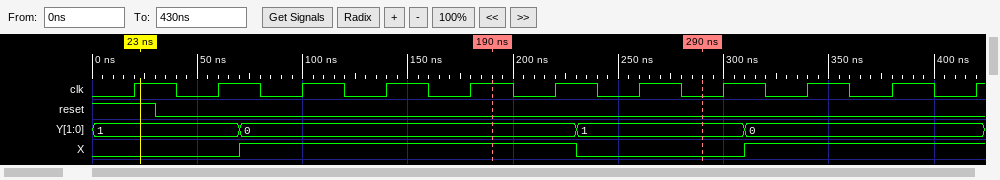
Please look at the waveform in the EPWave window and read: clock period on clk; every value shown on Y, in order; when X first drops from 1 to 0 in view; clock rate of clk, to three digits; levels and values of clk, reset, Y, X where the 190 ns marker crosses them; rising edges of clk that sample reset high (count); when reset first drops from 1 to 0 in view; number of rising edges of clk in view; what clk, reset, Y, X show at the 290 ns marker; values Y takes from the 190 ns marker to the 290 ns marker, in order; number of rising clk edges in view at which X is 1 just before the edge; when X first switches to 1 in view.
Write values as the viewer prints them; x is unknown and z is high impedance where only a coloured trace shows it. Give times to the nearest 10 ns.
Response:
40 ns
1, 0, 1, 0
230 ns
25.0 MHz
clk=1, reset=0, Y=0, X=1
1
30 ns
11
clk=0, reset=0, Y=1, X=0
0, 1
7
70 ns
